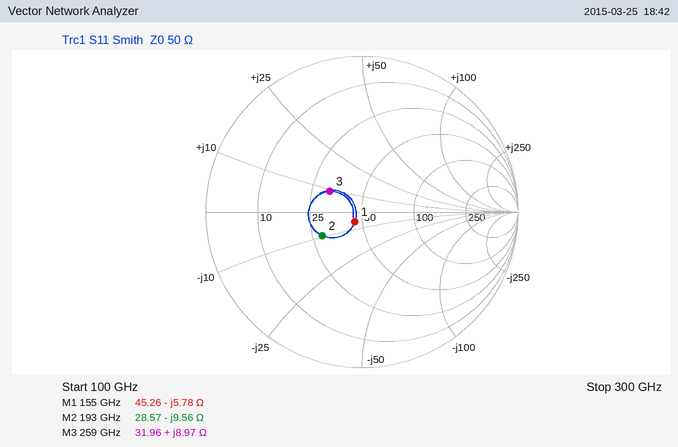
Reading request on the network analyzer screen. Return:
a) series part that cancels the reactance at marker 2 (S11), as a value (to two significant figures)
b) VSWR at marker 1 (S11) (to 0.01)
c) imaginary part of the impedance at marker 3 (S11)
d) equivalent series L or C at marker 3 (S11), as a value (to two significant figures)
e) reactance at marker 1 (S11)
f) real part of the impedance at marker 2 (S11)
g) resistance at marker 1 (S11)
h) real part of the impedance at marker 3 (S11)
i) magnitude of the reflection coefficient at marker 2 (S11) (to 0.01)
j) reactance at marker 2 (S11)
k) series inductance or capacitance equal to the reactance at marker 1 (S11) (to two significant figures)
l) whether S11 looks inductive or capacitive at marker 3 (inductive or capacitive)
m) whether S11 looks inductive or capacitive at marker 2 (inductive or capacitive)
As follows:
7.9 pH
1.17
+8.97 Ω
5.5 pH
-5.78 Ω
28.57 Ω
45.26 Ω
31.96 Ω
0.30
-9.56 Ω
180 fF
inductive
capacitive
